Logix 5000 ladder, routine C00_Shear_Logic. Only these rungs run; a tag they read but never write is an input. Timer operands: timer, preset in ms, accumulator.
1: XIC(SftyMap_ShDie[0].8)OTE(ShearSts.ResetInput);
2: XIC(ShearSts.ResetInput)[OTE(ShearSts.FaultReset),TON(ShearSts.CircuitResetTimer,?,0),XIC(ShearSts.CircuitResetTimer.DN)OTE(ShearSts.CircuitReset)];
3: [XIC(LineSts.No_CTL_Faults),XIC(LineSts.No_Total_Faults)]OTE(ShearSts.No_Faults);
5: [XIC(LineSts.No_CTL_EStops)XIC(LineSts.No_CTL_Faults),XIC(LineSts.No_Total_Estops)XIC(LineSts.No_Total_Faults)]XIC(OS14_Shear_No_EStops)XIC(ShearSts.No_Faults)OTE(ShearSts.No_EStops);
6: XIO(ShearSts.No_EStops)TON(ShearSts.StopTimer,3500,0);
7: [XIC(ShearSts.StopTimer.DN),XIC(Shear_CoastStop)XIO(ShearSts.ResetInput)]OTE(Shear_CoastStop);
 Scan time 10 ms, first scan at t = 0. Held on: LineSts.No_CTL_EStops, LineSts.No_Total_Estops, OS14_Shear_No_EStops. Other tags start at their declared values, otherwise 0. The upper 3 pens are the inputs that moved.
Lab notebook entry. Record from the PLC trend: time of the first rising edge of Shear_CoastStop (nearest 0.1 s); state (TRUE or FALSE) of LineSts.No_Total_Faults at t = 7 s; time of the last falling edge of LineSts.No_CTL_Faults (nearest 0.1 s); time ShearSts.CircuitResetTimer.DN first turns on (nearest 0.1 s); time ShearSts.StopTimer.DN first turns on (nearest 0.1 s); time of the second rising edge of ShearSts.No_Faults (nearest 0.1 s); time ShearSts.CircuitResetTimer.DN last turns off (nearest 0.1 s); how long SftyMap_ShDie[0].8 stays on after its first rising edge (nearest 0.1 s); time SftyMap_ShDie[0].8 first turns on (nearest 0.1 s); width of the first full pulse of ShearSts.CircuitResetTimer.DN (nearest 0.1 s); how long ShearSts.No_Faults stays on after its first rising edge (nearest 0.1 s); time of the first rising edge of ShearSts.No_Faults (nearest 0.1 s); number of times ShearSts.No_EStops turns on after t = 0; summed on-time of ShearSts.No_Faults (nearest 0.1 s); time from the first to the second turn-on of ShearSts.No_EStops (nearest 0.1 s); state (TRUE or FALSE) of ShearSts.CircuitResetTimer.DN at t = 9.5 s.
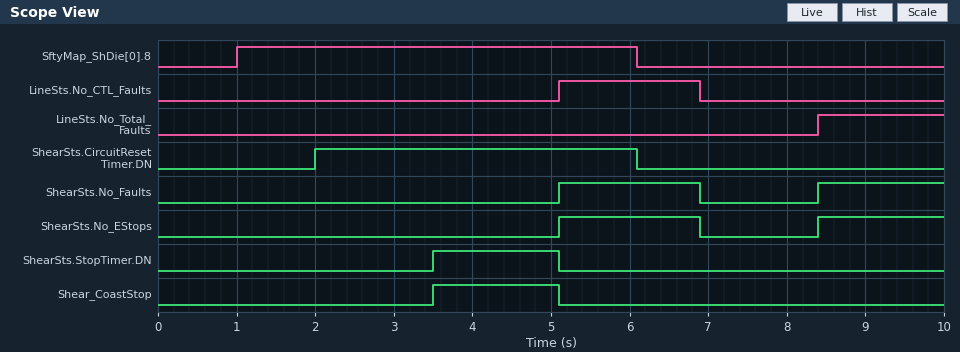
3.5 s
FALSE
6.9 s
2.0 s
3.5 s
8.4 s
6.1 s
5.1 s
1.0 s
4.1 s
1.8 s
5.1 s
2
3.4 s
3.3 s
FALSE
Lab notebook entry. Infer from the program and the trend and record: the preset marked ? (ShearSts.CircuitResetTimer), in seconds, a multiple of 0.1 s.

1.0 s
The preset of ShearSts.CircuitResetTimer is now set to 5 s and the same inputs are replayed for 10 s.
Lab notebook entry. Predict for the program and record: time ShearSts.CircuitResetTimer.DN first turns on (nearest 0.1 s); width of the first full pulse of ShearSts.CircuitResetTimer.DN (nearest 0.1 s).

6.0 s
0.1 s
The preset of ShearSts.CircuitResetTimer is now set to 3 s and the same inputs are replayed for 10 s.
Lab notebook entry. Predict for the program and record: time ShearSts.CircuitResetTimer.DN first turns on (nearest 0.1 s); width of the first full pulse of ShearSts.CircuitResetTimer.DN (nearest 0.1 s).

4.0 s
2.1 s
